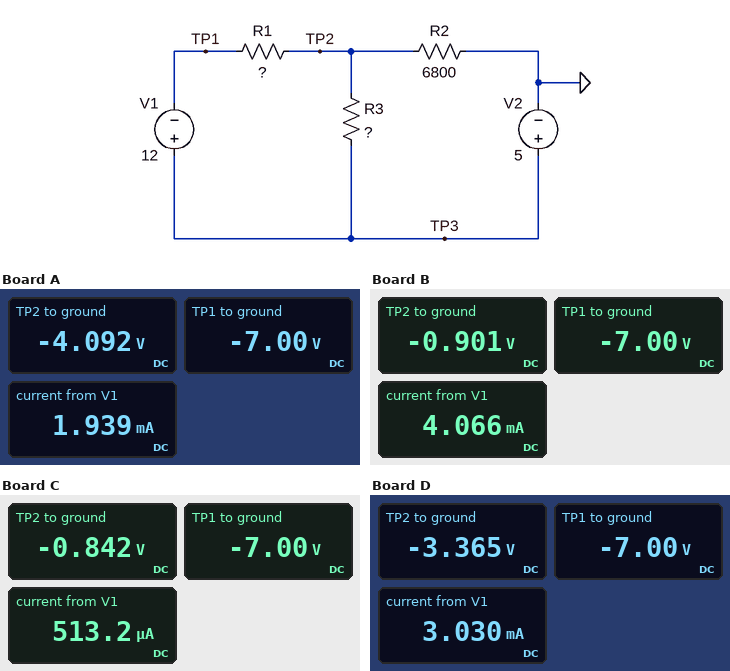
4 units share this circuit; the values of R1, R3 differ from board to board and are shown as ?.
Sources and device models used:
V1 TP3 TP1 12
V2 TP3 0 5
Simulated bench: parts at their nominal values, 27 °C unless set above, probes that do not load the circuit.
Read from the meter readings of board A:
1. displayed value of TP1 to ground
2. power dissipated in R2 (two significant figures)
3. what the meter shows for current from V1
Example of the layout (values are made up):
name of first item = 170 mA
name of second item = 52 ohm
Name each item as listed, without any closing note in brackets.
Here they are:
displayed value of TP1 to ground = -7.00 V
power dissipated in R2 = 2.5 mW
what the meter shows for current from V1 = 1.939 mA
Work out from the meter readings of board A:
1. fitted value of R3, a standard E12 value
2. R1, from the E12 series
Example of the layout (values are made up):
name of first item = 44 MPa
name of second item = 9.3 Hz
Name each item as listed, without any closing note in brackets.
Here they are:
fitted value of R3, a standard E12 value = 6.8 kΩ
R1, from the E12 series = 1.5 kΩ
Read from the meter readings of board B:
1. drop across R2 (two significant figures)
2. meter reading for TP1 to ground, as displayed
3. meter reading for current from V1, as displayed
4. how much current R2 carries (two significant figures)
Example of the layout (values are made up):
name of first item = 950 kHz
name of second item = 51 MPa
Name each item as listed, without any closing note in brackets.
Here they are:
drop across R2 = 900 mV
meter reading for TP1 to ground, as displayed = -7.00 V
meter reading for current from V1, as displayed = 4.066 mA
how much current R2 carries = 130 µA
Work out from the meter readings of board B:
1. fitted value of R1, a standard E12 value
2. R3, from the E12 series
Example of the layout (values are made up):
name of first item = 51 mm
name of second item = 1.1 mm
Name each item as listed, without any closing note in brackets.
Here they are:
fitted value of R1, a standard E12 value = 1.5 kΩ
R3, from the E12 series = 1.5 kΩ
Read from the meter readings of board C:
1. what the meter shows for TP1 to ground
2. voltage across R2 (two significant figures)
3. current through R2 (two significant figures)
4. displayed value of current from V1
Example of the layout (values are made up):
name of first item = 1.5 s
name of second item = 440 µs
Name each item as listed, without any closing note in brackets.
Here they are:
what the meter shows for TP1 to ground = -7.00 V
voltage across R2 = 840 mV
current through R2 = 120 µA
displayed value of current from V1 = 513.2 µA
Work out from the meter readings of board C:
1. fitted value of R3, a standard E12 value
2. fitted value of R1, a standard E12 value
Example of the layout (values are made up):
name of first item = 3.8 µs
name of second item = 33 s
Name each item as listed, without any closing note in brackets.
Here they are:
fitted value of R3, a standard E12 value = 15 kΩ
fitted value of R1, a standard E12 value = 12 kΩ
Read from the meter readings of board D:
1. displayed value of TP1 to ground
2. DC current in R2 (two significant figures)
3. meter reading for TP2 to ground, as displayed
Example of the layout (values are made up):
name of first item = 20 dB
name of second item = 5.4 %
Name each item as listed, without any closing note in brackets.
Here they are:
displayed value of TP1 to ground = -7.00 V
DC current in R2 = 490 µA
meter reading for TP2 to ground, as displayed = -3.365 V
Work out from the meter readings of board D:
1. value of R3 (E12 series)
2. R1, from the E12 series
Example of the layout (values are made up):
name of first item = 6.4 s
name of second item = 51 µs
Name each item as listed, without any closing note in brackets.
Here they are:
value of R3 = 3.3 kΩ
R1, from the E12 series = 1.2 kΩ
